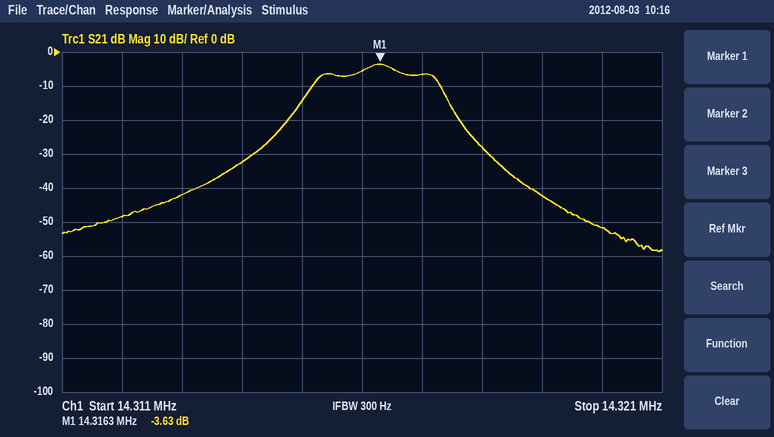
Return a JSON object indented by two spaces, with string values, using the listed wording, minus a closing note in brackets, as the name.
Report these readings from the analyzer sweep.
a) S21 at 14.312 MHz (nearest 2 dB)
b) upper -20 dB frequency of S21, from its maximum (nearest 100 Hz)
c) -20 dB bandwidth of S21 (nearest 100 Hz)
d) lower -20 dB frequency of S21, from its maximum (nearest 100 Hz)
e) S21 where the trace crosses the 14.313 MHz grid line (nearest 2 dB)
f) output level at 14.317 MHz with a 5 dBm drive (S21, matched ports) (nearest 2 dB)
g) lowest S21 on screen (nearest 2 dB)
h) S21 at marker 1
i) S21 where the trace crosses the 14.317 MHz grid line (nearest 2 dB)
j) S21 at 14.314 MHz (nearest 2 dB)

{
  "S21 at 14.312 MHz": "-48 dB",
  "upper -20 dB frequency of S21, from its maximum": "14.3178 MHz",
  "-20 dB bandwidth of S21": "3.2 kHz",
  "lower -20 dB frequency of S21, from its maximum": "14.3146 MHz",
  "S21 where the trace crosses the 14.313 MHz grid line": "-42 dB",
  "output level at 14.317 MHz with a 5 dBm drive (S21, matched ports)": "-2 dBm",
  "lowest S21 on screen": "-58 dB",
  "S21 at marker 1": "-3.63 dB",
  "S21 where the trace crosses the 14.317 MHz grid line": "-6 dB",
  "S21 at 14.314 MHz": "-32 dB"
}
